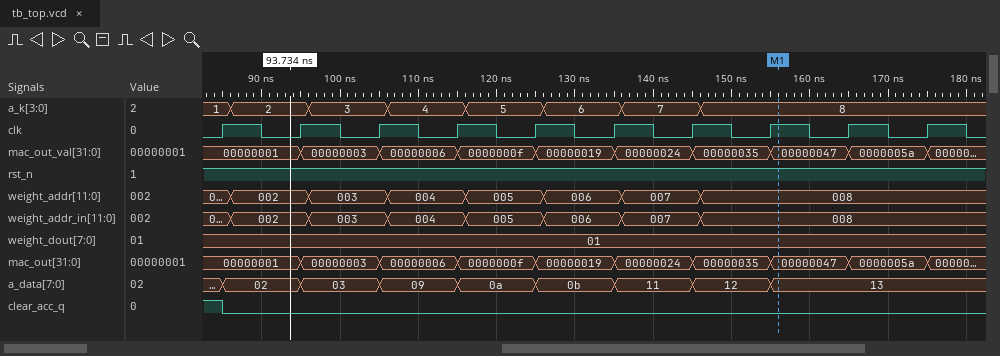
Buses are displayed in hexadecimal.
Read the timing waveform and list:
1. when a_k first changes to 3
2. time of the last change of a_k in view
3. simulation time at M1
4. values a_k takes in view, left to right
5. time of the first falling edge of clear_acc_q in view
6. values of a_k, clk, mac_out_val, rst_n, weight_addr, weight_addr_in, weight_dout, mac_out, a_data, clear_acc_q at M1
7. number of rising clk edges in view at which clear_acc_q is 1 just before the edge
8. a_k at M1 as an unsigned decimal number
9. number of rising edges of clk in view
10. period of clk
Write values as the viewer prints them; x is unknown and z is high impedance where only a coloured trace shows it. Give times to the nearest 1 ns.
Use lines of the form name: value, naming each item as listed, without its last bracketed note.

when a_k first changes to 3: 96 ns
time of the last change of a_k in view: 146 ns
simulation time at M1: 156 ns
values a_k takes in view, left to right: 1, 2, 3, 4, 5, 6, 7, 8
time of the first falling edge of clear_acc_q in view: 85 ns
values of a_k, clk, mac_out_val, rst_n, weight_addr, weight_addr_in, weight_dout, mac_out, a_data, clear_acc_q at M1: a_k=8, clk=1, mac_out_val=00000047, rst_n=1, weight_addr=008, weight_addr_in=008, weight_dout=01, mac_out=00000047, a_data=13, clear_acc_q=0
number of rising clk edges in view at which clear_acc_q is 1 just before the edge: 1
a_k at M1 as an unsigned decimal number: 8
number of rising edges of clk in view: 10
period of clk: 10 ns
